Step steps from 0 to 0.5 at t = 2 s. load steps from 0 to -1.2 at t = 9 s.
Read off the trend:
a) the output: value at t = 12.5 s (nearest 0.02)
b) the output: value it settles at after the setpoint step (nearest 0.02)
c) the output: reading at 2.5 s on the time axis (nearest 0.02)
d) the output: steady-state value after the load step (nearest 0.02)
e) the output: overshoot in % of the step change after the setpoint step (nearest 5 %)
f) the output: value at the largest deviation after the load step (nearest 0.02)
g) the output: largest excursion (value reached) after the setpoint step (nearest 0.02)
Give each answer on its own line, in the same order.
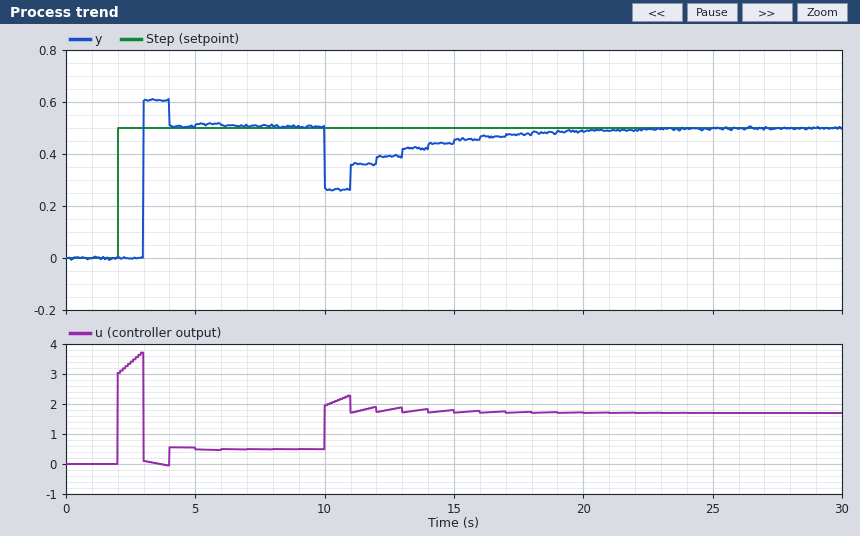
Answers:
0.40
0.50
0.00
0.50
20 %
0.26
0.60
